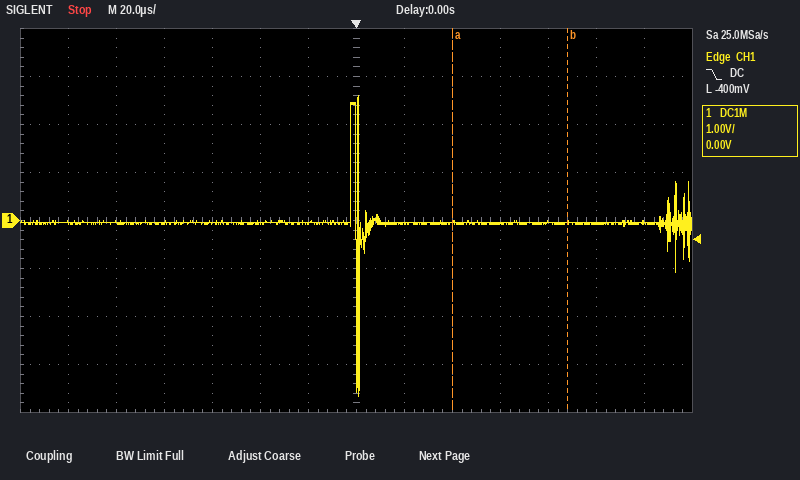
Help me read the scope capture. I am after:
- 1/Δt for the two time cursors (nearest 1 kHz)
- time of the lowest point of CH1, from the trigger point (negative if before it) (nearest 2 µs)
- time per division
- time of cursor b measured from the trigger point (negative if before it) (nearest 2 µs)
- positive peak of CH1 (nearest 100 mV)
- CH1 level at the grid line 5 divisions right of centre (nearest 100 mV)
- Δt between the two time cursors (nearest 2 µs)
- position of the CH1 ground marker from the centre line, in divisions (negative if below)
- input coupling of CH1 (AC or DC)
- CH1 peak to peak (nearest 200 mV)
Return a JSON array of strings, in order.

["21 kHz", "0 µs", "20 µs", "+88 µs", "2.6 V", "-100 mV", "48 µs", "0.0 div", "DC", "6.2 V"]
